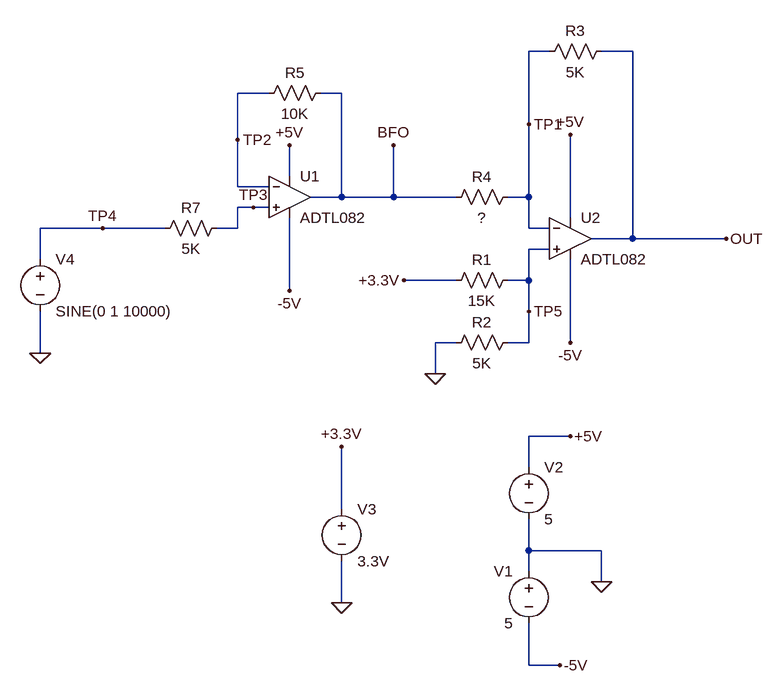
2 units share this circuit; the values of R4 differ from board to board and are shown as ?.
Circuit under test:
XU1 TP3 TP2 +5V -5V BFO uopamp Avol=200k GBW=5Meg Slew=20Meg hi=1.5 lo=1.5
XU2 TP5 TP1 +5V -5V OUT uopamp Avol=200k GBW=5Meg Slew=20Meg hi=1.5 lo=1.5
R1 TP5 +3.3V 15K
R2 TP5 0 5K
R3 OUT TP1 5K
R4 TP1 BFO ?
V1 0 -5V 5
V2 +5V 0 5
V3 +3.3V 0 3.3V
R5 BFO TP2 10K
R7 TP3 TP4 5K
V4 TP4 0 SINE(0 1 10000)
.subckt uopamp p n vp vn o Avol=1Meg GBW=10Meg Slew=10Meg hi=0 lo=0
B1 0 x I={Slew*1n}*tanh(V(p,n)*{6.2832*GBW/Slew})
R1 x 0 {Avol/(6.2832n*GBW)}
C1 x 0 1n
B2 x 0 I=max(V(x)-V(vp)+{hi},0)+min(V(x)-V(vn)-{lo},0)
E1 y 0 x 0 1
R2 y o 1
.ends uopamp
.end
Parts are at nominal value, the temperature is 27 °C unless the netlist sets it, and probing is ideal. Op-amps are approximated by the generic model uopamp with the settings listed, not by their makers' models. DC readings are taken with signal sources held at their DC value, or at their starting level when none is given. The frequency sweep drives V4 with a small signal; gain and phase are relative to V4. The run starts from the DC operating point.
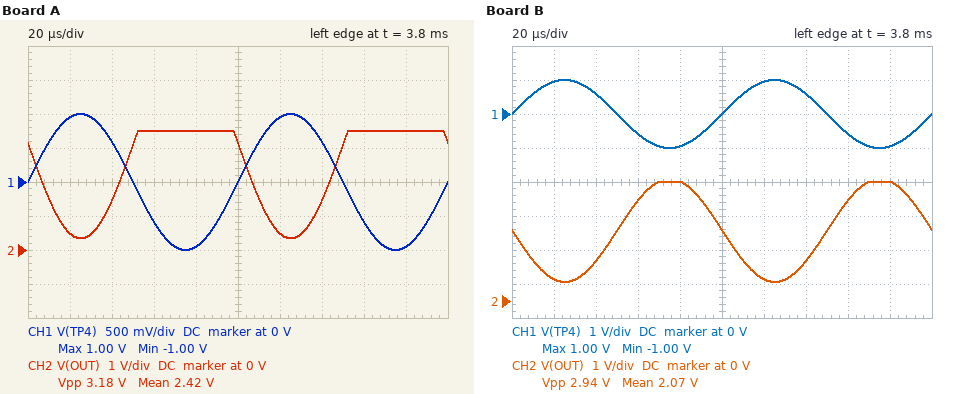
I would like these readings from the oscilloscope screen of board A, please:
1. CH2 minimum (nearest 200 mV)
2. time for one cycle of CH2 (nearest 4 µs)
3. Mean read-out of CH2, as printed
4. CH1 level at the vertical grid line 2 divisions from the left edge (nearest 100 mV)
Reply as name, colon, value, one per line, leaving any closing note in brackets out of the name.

CH2 minimum: 400 mV
time for one cycle of CH2: 100 µs
Mean read-out of CH2, as printed: 2.42 V
CH1 level at the vertical grid line 2 divisions from the left edge: 600 mV
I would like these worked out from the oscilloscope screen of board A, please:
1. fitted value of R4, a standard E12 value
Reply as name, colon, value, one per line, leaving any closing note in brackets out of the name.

fitted value of R4, a standard E12 value: 1.8 kΩ
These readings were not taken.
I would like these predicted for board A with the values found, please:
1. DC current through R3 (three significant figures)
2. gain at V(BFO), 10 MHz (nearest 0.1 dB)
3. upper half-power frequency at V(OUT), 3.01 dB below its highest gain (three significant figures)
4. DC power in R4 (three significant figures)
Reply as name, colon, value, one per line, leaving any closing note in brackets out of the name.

DC current through R3: 458 µA
gain at V(BFO), 10 MHz: -7.0 dB
upper half-power frequency at V(OUT), 3.01 dB below its highest gain: 1.24 MHz
DC power in R4: 378 µW
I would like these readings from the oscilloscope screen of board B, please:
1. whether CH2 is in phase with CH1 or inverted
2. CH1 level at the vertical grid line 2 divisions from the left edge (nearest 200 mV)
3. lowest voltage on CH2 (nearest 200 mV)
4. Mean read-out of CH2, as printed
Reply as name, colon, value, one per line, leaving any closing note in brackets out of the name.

whether CH2 is in phase with CH1 or inverted: inverted
CH1 level at the vertical grid line 2 divisions from the left edge: 600 mV
lowest voltage on CH2: 600 mV
Mean read-out of CH2, as printed: 2.07 V
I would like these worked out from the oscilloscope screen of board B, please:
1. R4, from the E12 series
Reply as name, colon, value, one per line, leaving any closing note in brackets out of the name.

R4, from the E12 series: 3.3 kΩ
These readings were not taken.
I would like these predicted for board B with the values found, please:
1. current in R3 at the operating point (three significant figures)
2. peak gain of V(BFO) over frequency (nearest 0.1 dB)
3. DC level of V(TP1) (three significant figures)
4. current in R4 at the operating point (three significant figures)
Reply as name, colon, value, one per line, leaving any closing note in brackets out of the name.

current in R3 at the operating point: 250 µA
peak gain of V(BFO) over frequency: 0 dB
DC level of V(TP1): 825 mV
current in R4 at the operating point: 250 µA
